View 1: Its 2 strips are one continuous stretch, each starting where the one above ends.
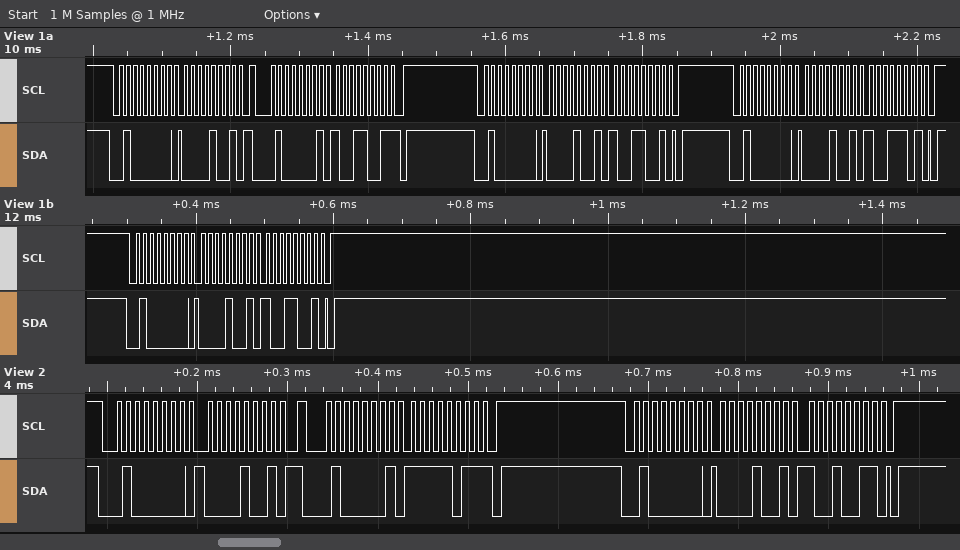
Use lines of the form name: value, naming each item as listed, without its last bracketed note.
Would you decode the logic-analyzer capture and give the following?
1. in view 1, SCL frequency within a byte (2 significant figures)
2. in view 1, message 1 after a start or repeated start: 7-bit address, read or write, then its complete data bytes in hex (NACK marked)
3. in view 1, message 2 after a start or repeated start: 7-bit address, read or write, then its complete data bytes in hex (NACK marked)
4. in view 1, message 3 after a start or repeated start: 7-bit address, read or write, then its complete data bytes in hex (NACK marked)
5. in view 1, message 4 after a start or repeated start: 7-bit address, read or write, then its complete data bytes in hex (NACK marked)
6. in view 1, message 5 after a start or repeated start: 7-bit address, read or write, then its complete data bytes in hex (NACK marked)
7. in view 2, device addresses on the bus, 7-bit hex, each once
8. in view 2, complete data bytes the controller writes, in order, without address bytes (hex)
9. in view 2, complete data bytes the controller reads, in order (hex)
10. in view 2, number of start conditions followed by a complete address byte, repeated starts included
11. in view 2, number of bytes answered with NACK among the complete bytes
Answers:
in view 1, SCL frequency within a byte: 100 kHz
in view 1, message 1 after a start or repeated start: 7-bit address, read or write, then its complete data bytes in hex: 0x20 write: 09
in view 1, message 2 after a start or repeated start: 7-bit address, read or write, then its complete data bytes in hex: 0x20 read: 99 NACK
in view 1, message 3 after a start or repeated start: 7-bit address, read or write, then its complete data bytes in hex: 0x20 write: 09 99
in view 1, message 4 after a start or repeated start: 7-bit address, read or write, then its complete data bytes in hex: 0x20 write: 09 9D
in view 1, message 5 after a start or repeated start: 7-bit address, read or write, then its complete data bytes in hex: 0x20 write: 09 99
in view 2, device addresses on the bus, 7-bit hex, each once: 0x20
in view 2, complete data bytes the controller writes, in order, without address bytes: 09 09 93
in view 2, complete data bytes the controller reads, in order: FB
in view 2, number of start conditions followed by a complete address byte, repeated starts included: 3
in view 2, number of bytes answered with NACK among the complete bytes: 1
